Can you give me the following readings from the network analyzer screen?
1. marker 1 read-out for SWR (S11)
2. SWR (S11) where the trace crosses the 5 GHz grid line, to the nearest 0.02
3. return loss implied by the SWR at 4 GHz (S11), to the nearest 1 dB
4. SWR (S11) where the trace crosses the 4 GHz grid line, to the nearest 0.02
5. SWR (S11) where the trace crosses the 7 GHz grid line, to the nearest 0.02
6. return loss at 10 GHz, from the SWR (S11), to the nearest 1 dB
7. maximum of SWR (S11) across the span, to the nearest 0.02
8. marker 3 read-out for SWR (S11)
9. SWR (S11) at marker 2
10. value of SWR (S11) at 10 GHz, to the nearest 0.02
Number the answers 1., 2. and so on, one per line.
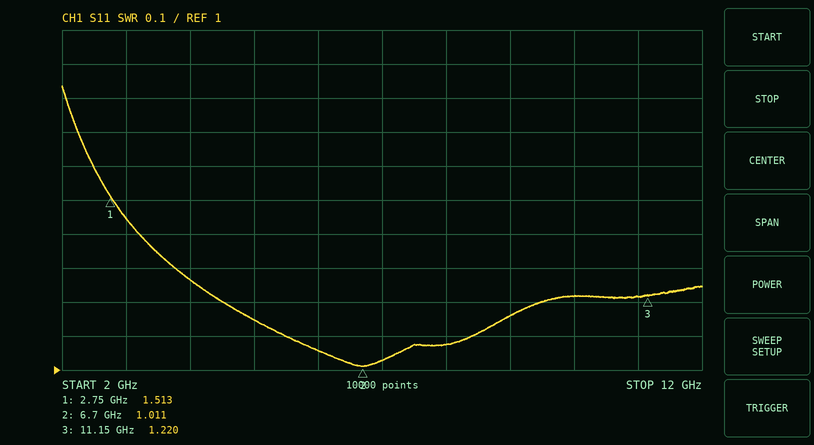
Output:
1. 1.513
2. 1.14
3. 19 dB
4. 1.26
5. 1.02
6. 20 dB
7. 1.84
8. 1.220
9. 1.011
10. 1.22
